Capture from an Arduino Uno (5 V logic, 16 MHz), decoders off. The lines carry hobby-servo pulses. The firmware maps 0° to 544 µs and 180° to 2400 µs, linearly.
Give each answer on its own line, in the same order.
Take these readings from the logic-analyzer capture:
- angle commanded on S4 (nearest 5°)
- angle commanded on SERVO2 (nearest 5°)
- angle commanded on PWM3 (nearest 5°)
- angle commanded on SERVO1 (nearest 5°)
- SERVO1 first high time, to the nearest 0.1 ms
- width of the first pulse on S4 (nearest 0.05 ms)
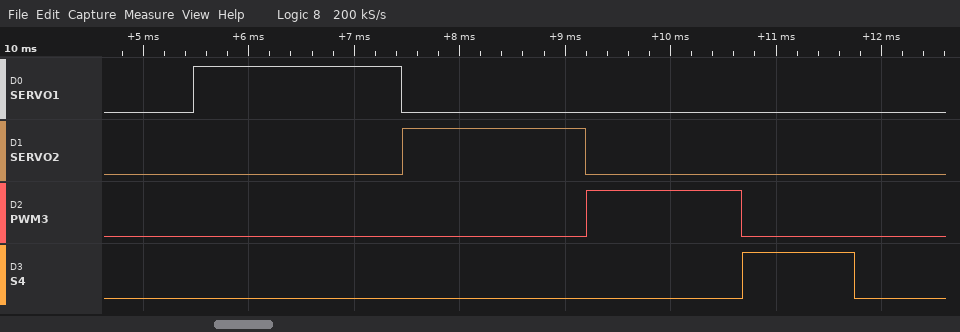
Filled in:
50°
115°
90°
140°
2.0 ms
1.05 ms
